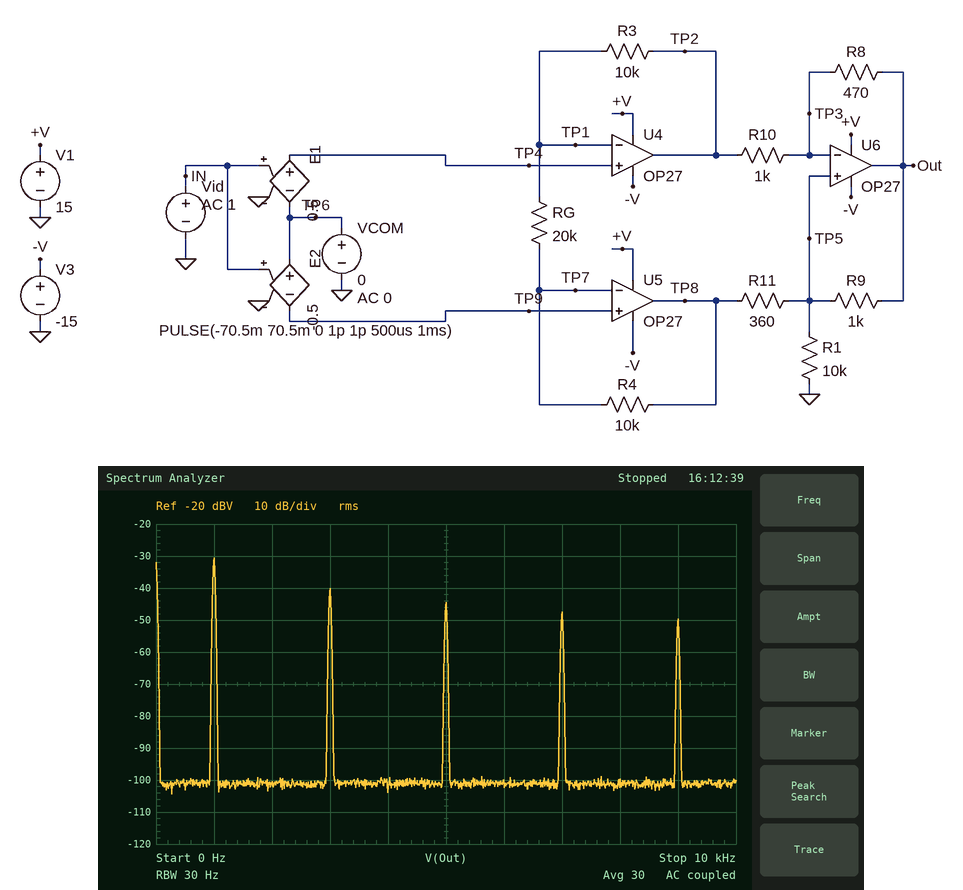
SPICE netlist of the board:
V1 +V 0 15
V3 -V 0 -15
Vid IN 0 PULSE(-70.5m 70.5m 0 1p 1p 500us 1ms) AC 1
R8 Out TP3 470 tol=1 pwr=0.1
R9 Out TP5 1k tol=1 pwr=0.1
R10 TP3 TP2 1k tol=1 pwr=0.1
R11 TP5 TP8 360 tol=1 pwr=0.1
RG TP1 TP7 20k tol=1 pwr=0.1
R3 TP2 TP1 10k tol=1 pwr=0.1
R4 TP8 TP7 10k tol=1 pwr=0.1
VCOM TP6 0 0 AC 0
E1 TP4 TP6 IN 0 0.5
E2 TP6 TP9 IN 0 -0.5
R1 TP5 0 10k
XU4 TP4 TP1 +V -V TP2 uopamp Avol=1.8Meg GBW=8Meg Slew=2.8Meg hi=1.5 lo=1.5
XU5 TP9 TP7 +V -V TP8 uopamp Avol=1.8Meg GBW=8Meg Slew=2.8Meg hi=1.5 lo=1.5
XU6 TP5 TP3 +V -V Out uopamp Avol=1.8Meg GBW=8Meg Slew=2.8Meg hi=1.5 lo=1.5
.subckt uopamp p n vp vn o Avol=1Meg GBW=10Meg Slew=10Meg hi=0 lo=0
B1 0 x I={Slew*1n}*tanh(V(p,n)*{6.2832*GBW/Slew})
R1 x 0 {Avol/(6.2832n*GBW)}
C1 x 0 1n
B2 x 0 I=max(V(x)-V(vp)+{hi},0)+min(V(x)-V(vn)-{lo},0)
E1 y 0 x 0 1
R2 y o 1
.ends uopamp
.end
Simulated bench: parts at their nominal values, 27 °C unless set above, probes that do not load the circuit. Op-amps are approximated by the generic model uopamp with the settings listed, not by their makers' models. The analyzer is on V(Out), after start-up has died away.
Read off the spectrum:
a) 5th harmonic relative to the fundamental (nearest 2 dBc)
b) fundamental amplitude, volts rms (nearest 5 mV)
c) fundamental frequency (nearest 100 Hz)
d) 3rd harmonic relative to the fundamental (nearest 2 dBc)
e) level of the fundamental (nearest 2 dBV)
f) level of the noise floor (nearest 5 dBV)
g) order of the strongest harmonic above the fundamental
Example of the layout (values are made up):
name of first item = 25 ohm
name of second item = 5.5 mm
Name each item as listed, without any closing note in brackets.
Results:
5th harmonic relative to the fundamental = -14 dBc
fundamental amplitude, volts rms = 30 mV
fundamental frequency = 1.0 kHz
3rd harmonic relative to the fundamental = -10 dBc
level of the fundamental = -30 dBV
level of the noise floor = -100 dBV
order of the strongest harmonic above the fundamental = 3
